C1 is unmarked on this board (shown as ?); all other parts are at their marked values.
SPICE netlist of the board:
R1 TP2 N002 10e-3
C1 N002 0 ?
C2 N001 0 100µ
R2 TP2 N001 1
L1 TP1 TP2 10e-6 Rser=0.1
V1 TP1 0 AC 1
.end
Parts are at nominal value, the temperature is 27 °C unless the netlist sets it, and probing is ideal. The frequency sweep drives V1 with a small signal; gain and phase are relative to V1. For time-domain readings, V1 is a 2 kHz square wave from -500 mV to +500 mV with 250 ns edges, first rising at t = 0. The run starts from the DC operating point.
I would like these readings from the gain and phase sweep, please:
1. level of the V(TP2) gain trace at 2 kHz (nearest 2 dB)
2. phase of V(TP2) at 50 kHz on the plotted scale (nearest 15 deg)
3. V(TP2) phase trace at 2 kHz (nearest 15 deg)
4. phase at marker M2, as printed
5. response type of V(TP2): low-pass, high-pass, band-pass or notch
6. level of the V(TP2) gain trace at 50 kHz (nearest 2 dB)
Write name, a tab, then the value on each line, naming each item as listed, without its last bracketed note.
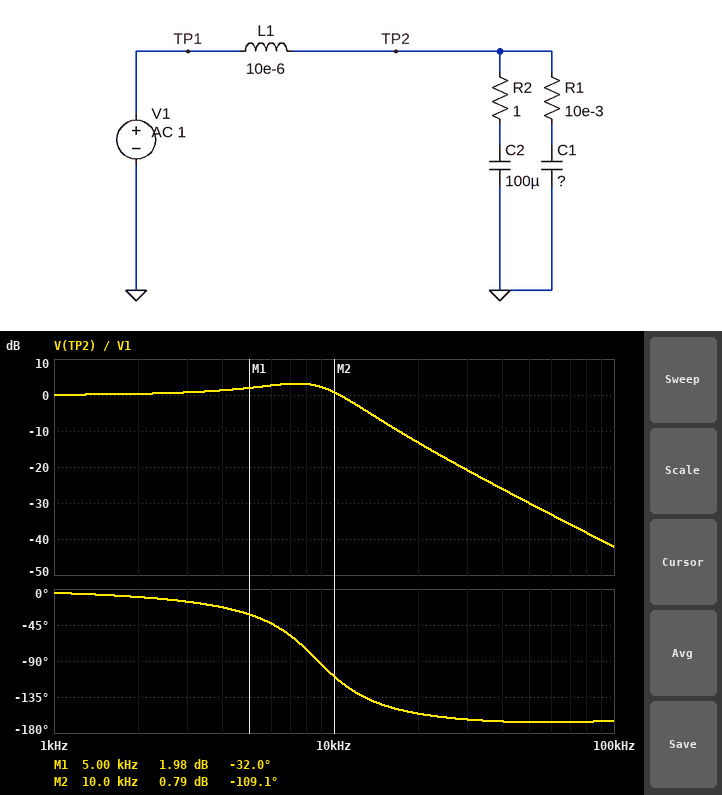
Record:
level of the V(TP2) gain trace at 2 kHz	0 dB
phase of V(TP2) at 50 kHz on the plotted scale	-165 deg
V(TP2) phase trace at 2 kHz	-15 deg
phase at marker M2, as printed	-109.1 deg
response type of V(TP2): low-pass, high-pass, band-pass or notch	low-pass
level of the V(TP2) gain trace at 50 kHz	-30 dB
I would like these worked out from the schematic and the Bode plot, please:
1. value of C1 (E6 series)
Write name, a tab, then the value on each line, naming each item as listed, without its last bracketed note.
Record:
value of C1	33 µF
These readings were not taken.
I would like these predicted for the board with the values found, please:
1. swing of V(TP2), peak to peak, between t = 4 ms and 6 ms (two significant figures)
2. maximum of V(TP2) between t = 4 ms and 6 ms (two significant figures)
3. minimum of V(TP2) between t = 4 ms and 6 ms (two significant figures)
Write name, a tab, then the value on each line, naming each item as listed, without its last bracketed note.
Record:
swing of V(TP2), peak to peak, between t = 4 ms and 6 ms	1.6 V
maximum of V(TP2) between t = 4 ms and 6 ms	780 mV
minimum of V(TP2) between t = 4 ms and 6 ms	-780 mV
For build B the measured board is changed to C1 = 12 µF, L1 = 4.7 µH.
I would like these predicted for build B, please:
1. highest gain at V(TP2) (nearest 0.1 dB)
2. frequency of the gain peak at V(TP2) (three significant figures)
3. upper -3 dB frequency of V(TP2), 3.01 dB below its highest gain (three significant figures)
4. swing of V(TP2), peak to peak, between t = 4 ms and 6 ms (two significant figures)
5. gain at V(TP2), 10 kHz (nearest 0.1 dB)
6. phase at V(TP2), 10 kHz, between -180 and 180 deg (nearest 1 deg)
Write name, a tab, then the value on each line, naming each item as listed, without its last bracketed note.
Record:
highest gain at V(TP2)	2.4 dB
frequency of the gain peak at V(TP2)	18.1 kHz
upper -3 dB frequency of V(TP2), 3.01 dB below its highest gain	25.8 kHz
swing of V(TP2), peak to peak, between t = 4 ms and 6 ms	1.4 V
gain at V(TP2), 10 kHz	0.8 dB
phase at V(TP2), 10 kHz, between -180 and 180 deg	-25 deg
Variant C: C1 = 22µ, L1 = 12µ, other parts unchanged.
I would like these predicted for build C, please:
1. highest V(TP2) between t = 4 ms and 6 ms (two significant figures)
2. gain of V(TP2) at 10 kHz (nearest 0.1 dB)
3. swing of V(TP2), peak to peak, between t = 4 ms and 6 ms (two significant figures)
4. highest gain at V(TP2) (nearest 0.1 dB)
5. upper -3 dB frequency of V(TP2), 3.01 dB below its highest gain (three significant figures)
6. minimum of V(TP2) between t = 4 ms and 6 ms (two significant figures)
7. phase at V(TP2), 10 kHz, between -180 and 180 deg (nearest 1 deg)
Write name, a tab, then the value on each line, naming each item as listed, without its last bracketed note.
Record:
highest V(TP2) between t = 4 ms and 6 ms	730 mV
gain of V(TP2) at 10 kHz	0.9 dB
swing of V(TP2), peak to peak, between t = 4 ms and 6 ms	1.5 V
highest gain at V(TP2)	2.2 dB
upper -3 dB frequency of V(TP2), 3.01 dB below its highest gain	11.4 kHz
minimum of V(TP2) between t = 4 ms and 6 ms	-730 mV
phase at V(TP2), 10 kHz, between -180 and 180 deg	-94 deg
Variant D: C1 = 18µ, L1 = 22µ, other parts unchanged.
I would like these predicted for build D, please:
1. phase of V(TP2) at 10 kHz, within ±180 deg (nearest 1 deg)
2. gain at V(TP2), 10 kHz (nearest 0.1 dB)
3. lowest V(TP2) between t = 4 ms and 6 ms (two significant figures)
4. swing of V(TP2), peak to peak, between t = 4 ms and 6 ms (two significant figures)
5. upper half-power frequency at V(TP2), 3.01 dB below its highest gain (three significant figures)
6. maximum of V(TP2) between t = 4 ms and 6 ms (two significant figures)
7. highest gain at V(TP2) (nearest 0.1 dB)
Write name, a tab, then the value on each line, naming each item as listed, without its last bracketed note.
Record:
phase of V(TP2) at 10 kHz, within ±180 deg	-114 deg
gain at V(TP2), 10 kHz	-4.3 dB
lowest V(TP2) between t = 4 ms and 6 ms	-680 mV
swing of V(TP2), peak to peak, between t = 4 ms and 6 ms	1.4 V
upper half-power frequency at V(TP2), 3.01 dB below its highest gain	8.11 kHz
maximum of V(TP2) between t = 4 ms and 6 ms	680 mV
highest gain at V(TP2)	1.4 dB
